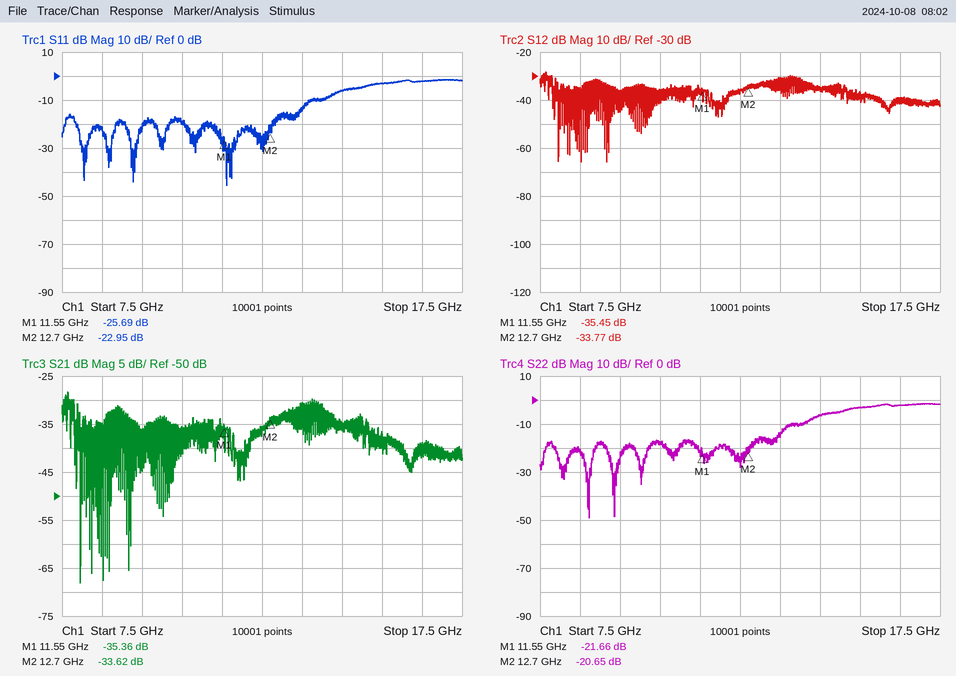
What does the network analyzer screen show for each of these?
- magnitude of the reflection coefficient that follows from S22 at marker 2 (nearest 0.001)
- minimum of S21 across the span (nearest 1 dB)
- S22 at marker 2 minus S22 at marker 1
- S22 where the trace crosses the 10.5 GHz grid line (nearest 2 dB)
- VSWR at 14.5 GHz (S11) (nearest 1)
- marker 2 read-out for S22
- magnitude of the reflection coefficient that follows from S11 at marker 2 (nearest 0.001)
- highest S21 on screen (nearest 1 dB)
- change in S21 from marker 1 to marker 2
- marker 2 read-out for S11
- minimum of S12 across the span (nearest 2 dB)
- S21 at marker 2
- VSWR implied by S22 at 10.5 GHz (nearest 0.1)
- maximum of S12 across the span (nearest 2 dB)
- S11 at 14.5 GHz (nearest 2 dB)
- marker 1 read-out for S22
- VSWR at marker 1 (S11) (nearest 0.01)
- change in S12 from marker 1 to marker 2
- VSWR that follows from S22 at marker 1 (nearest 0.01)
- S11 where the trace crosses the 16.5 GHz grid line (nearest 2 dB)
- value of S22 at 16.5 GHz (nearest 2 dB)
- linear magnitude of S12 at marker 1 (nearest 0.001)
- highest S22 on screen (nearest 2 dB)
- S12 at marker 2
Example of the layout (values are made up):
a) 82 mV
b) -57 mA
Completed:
a) 0.093
b) -68 dB
c) 1.01 dB
d) -18 dB
e) 3
f) -20.65 dB
g) 0.071
h) -28 dB
i) 1.74 dB
j) -22.95 dB
k) -66 dB
l) -33.62 dB
m) 1.3
n) -28 dB
o) -6 dB
p) -21.66 dB
q) 1.11
r) 1.68 dB
s) 1.18
t) -2 dB
u) -2 dB
v) 0.017
w) -2 dB
x) -33.77 dB
